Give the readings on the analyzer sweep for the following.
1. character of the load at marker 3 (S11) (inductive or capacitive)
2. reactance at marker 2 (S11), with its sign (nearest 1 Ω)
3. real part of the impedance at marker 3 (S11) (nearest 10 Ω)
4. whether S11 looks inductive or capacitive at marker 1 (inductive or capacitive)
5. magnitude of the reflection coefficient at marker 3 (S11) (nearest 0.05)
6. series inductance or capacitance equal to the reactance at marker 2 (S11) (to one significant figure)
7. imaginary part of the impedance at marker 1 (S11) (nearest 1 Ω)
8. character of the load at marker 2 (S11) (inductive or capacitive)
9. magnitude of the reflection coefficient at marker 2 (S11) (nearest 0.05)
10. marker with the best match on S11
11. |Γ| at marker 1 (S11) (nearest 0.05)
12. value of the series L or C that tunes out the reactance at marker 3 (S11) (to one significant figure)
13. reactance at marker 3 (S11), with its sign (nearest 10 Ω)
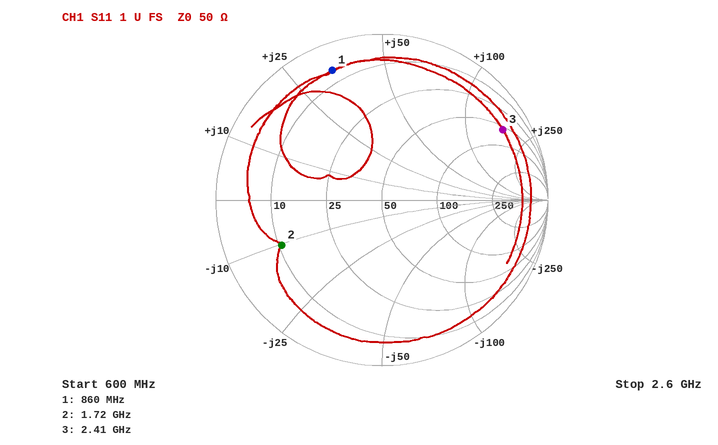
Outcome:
inductive
-10 Ω
60 Ω
inductive
0.85
9 pF
+34 Ω
capacitive
0.65
marker 2
0.85
400 fF
+170 Ω
